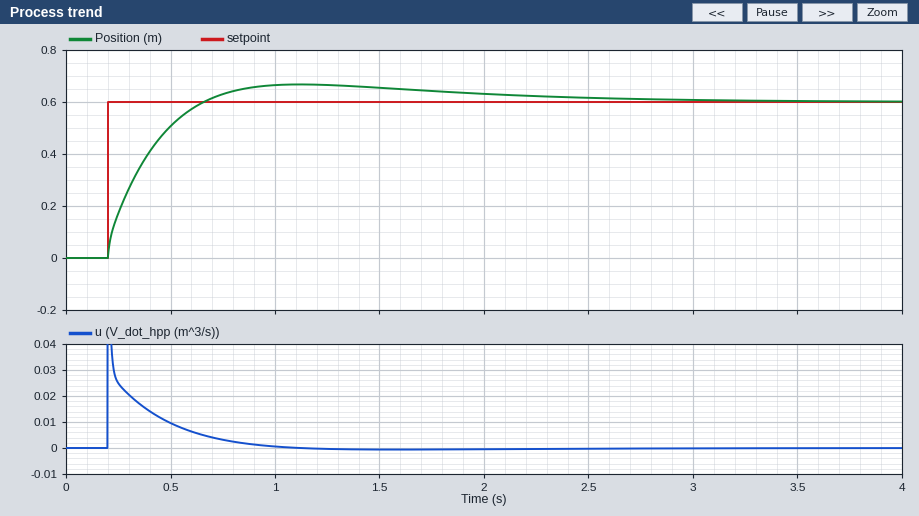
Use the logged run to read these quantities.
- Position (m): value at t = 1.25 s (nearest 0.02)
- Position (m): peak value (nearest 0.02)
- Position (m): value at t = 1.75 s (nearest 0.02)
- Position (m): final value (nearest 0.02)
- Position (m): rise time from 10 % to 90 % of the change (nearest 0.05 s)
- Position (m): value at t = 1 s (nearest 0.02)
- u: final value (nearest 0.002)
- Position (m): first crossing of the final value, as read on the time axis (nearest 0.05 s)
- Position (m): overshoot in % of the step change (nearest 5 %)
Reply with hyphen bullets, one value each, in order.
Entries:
- 0.66
- 0.66
- 0.64
- 0.60
- 0.35 s
- 0.66
- 0.000
- 0.65 s
- 10 %
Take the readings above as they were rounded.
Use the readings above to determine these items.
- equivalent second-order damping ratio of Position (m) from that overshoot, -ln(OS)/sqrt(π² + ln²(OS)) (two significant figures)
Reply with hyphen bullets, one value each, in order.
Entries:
- 0.59
